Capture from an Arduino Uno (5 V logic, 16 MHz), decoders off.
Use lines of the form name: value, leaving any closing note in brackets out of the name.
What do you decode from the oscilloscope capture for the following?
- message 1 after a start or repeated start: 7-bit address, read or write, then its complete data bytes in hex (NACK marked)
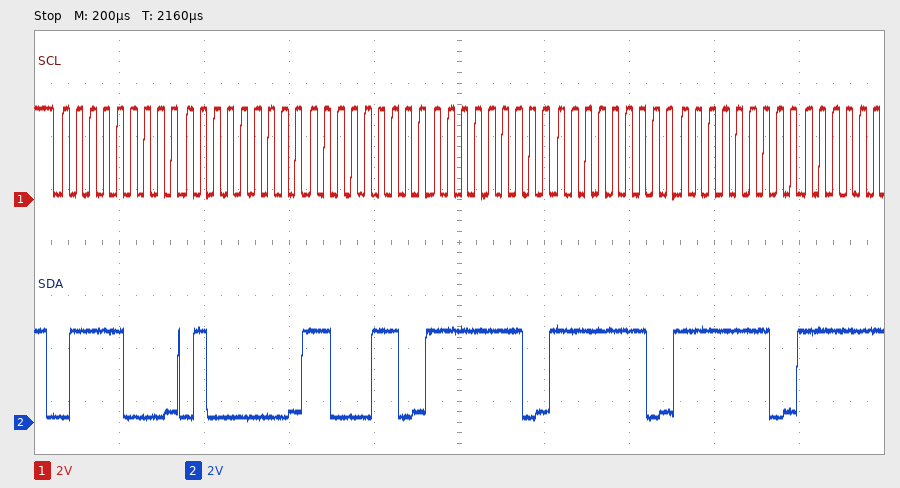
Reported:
message 1 after a start or repeated start: 7-bit address, read or write, then its complete data bytes in hex: 0x3C write: 40 C6 FE FE FE
